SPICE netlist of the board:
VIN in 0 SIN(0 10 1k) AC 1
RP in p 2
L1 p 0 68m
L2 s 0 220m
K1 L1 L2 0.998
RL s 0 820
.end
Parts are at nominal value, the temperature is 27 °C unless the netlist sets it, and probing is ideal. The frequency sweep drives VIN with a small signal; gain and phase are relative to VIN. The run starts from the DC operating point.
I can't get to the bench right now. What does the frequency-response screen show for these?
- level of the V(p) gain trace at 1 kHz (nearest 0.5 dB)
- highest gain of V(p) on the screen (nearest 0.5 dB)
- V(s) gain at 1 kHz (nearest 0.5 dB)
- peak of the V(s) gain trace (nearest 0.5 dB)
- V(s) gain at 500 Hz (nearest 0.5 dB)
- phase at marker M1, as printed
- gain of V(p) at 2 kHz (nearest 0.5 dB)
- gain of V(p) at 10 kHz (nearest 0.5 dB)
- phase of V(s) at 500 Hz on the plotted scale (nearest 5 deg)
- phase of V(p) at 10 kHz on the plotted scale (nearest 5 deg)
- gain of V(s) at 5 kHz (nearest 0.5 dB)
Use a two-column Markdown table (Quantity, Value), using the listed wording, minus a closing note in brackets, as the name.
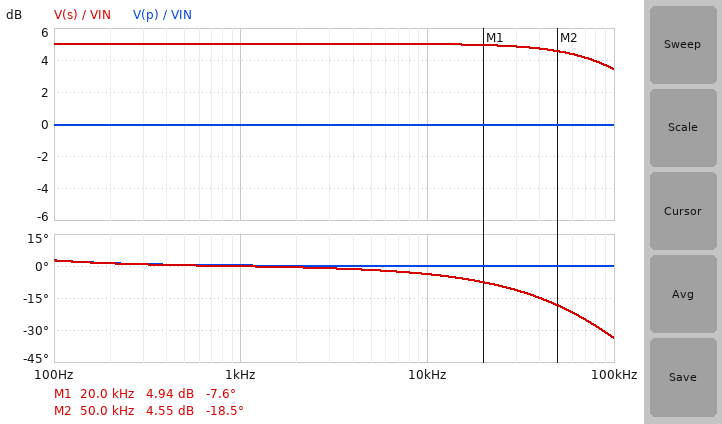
| Quantity | Value |
|---|---|
| level of the V(p) gain trace at 1 kHz | 0 dB |
| highest gain of V(p) on the screen | 0 dB |
| V(s) gain at 1 kHz | 5.0 dB |
| peak of the V(s) gain trace | 5.0 dB |
| V(s) gain at 500 Hz | 5.0 dB |
| phase at marker M1, as printed | -7.6 deg |
| gain of V(p) at 2 kHz | 0 dB |
| gain of V(p) at 10 kHz | 0 dB |
| phase of V(s) at 500 Hz on the plotted scale | 0 deg |
| phase of V(p) at 10 kHz on the plotted scale | 0 deg |
| gain of V(s) at 5 kHz | 5.0 dB |
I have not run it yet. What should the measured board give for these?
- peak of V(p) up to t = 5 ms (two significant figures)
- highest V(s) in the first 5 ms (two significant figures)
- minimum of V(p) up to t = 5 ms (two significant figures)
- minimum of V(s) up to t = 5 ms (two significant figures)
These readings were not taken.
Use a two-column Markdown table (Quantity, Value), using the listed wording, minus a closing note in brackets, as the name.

| Quantity | Value |
|---|---|
| peak of V(p) up to t = 5 ms | 9.9 V |
| highest V(s) in the first 5 ms | 18 V |
| minimum of V(p) up to t = 5 ms | -10 V |
| minimum of V(s) up to t = 5 ms | -18 V |
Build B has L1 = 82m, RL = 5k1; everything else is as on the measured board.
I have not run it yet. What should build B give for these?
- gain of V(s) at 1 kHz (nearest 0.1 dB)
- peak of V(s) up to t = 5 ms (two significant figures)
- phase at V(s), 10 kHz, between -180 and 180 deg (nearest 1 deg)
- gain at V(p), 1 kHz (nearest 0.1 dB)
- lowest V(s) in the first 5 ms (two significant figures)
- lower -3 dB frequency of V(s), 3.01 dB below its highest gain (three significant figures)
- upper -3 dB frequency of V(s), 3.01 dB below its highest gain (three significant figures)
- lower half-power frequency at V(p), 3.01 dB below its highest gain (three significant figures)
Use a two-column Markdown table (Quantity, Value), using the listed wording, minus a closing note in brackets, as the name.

| Quantity | Value |
|---|---|
| gain of V(s) at 1 kHz | 4.3 dB |
| peak of V(s) up to t = 5 ms | 16 V |
| phase at V(s), 10 kHz, between -180 and 180 deg | -1 deg |
| gain at V(p), 1 kHz | 0 dB |
| lowest V(s) in the first 5 ms | -16 V |
| lower -3 dB frequency of V(s), 3.01 dB below its highest gain | 3.88 Hz |
| upper -3 dB frequency of V(s), 3.01 dB below its highest gain | 924 kHz |
| lower half-power frequency at V(p), 3.01 dB below its highest gain | 3.89 Hz |
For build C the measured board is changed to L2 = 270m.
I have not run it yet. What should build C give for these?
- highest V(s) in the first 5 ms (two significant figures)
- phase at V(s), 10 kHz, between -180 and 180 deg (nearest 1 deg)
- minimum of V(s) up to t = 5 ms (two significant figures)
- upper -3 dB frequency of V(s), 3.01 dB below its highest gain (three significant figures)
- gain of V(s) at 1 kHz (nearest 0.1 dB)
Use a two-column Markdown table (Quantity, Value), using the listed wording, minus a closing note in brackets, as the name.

| Quantity | Value |
|---|---|
| highest V(s) in the first 5 ms | 20 V |
| phase at V(s), 10 kHz, between -180 and 180 deg | -5 deg |
| minimum of V(s) up to t = 5 ms | -20 V |
| upper -3 dB frequency of V(s), 3.01 dB below its highest gain | 122 kHz |
| gain of V(s) at 1 kHz | 5.9 dB |
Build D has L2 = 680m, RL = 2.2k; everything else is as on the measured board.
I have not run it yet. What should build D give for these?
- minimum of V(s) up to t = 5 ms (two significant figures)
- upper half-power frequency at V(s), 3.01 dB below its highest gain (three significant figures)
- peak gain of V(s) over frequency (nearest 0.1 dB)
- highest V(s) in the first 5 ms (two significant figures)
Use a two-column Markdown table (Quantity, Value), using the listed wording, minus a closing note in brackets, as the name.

| Quantity | Value |
|---|---|
| minimum of V(s) up to t = 5 ms | -31 V |
| upper half-power frequency at V(s), 3.01 dB below its highest gain | 130 kHz |
| peak gain of V(s) over frequency | 9.9 dB |
| highest V(s) in the first 5 ms | 31 V |
